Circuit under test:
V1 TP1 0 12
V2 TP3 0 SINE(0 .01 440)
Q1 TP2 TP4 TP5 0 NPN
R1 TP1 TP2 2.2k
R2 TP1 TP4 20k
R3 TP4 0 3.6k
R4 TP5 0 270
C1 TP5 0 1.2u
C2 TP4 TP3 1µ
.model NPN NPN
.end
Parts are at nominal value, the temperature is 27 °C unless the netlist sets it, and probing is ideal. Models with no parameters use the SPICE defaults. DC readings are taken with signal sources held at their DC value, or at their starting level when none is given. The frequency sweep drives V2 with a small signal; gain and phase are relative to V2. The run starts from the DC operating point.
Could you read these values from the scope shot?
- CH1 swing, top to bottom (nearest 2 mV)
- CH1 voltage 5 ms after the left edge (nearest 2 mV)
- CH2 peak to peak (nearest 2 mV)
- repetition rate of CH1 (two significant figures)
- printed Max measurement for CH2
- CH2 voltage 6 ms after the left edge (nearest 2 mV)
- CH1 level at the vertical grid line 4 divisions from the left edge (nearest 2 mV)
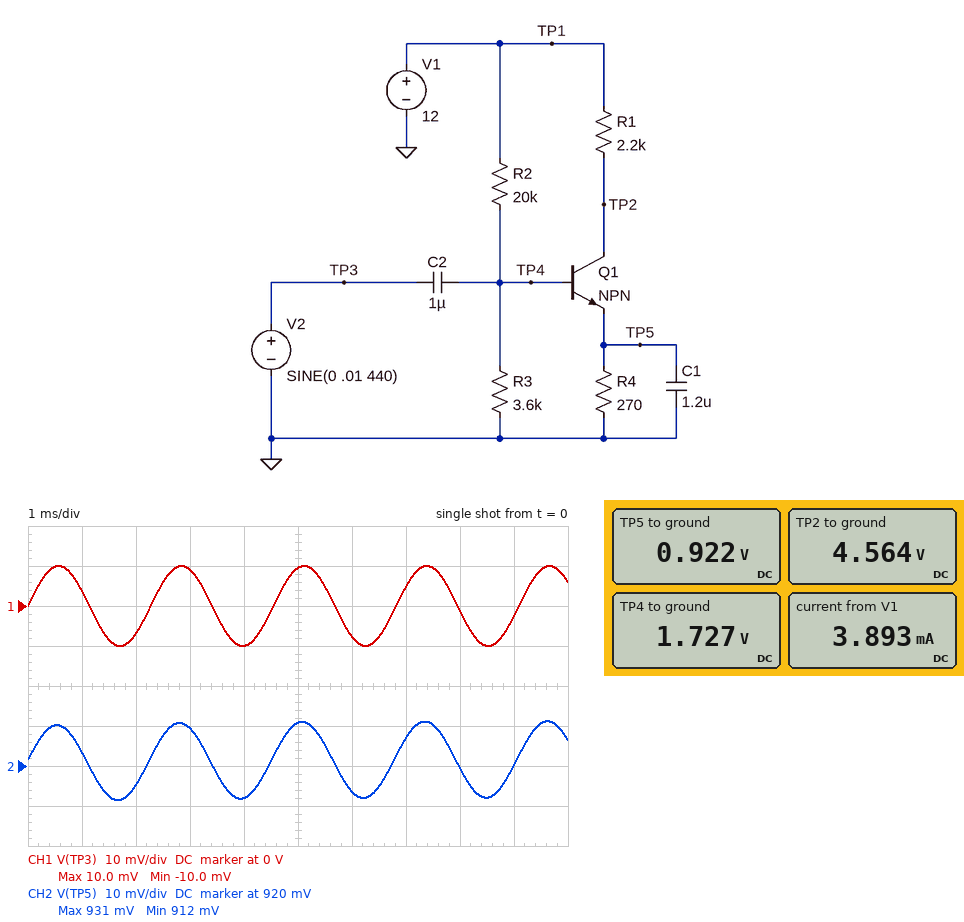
20 mV
10 mV
20 mV
440 Hz
931 mV
914 mV
-10 mV
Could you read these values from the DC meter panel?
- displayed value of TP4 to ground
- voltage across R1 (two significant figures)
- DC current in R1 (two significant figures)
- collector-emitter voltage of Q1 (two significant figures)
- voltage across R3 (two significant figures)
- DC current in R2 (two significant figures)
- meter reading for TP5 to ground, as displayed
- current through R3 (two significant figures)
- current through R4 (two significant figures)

1.727 V
7.4 V
3.4 mA
3.6 V
1.7 V
510 µA
0.922 V
480 µA
3.4 mA
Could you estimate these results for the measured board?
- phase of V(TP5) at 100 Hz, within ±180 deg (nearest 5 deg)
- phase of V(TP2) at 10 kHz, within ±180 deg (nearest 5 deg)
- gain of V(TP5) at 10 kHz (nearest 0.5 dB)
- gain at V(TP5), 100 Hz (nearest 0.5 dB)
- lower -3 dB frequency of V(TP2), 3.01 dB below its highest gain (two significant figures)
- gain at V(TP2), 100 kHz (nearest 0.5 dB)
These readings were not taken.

30 deg
-120 deg
-1.5 dB
-1.5 dB
18 kHz
49.0 dB
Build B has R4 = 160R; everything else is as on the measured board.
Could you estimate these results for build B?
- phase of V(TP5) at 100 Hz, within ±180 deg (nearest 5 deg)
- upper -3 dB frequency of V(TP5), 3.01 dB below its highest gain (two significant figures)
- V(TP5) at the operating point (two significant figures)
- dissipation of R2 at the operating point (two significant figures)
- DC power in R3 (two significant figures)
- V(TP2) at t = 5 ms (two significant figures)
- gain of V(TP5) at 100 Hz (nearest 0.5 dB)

75 deg
30 kHz
810 mV
5.4 mW
740 µW
950 mV
-17.0 dB
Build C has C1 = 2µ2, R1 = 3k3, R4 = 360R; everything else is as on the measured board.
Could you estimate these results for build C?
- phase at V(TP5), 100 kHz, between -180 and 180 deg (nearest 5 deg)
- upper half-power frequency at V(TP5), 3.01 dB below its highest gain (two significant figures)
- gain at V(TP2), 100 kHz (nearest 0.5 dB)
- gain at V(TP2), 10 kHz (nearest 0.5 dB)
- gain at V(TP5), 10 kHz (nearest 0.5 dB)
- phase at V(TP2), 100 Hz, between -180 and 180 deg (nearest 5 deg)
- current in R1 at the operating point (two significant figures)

-85 deg
7.9 kHz
50.5 dB
48.5 dB
-4.5 dB
-125 deg
2.6 mA
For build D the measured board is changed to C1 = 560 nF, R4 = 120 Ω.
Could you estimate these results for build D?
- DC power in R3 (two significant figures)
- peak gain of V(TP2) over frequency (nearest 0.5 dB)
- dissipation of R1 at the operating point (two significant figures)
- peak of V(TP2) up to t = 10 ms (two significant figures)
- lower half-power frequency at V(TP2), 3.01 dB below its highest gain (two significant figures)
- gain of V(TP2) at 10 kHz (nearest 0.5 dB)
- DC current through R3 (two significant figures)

580 µW
30.0 dB
58 mW
750 mV
49 kHz
16.5 dB
400 µA
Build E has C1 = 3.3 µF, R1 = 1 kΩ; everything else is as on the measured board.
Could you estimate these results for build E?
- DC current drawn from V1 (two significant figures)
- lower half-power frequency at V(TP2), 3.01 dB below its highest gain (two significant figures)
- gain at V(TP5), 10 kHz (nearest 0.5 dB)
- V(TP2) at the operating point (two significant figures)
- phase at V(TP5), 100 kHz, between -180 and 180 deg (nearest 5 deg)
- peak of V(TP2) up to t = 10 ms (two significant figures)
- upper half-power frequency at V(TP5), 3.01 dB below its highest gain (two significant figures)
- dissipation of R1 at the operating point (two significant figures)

3.9 mA
6.7 kHz
-5.5 dB
8.6 V
-85 deg
8.7 V
6.9 kHz
11 mW
